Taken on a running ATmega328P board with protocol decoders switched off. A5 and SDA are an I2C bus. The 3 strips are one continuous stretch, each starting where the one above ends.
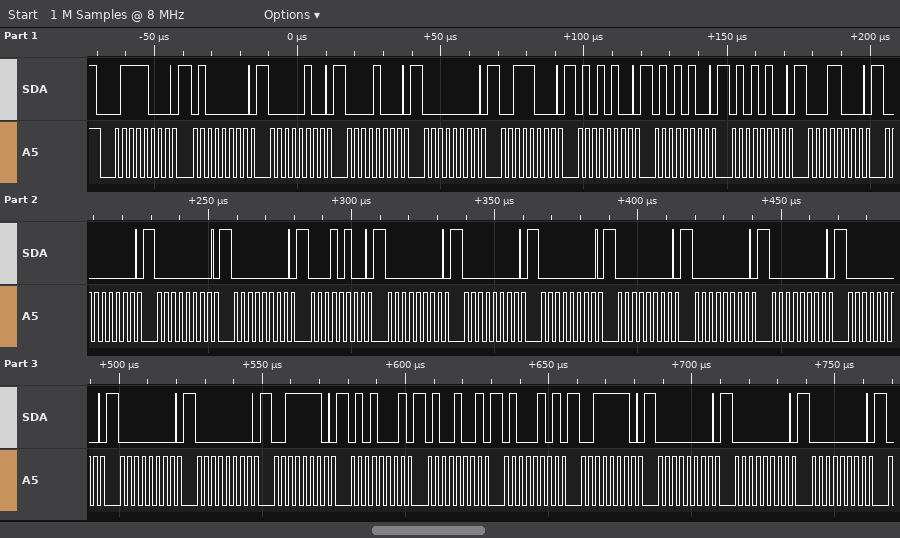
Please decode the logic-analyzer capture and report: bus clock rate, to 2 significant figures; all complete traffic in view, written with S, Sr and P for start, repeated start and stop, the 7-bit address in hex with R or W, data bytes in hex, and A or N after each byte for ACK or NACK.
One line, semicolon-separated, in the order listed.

400 kHz; S 3CW A 40 A 04 A 08 A 00 A 38 A 54 A 54 A 54 A 18 A 00 A 00 A 00 A 14 A 00 A 00 A 00 A 00 A 00 A 00 A 00 A 00 A 00 A 3E A 51 A 49 A 45 A 3E A 00 A 00 A 00 A
